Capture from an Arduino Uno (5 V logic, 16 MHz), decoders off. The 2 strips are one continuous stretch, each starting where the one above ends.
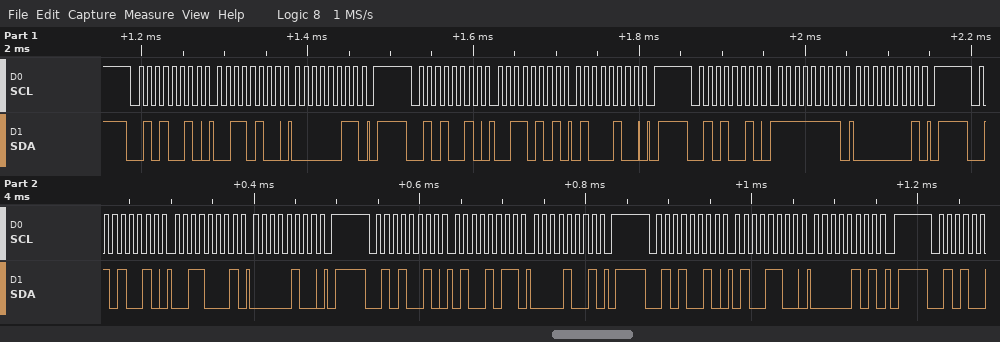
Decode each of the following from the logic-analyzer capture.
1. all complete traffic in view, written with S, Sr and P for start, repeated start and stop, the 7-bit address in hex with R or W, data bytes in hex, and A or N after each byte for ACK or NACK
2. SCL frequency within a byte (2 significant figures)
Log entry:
S 29W A 34 A 03 A P S 29W A 35 A 44 A P S 29W A FF A 01 A P S 29W A 31 A 04 A P S 29W A 4B A 09 A P S 29W A 4C A 05 A P
100 kHz
